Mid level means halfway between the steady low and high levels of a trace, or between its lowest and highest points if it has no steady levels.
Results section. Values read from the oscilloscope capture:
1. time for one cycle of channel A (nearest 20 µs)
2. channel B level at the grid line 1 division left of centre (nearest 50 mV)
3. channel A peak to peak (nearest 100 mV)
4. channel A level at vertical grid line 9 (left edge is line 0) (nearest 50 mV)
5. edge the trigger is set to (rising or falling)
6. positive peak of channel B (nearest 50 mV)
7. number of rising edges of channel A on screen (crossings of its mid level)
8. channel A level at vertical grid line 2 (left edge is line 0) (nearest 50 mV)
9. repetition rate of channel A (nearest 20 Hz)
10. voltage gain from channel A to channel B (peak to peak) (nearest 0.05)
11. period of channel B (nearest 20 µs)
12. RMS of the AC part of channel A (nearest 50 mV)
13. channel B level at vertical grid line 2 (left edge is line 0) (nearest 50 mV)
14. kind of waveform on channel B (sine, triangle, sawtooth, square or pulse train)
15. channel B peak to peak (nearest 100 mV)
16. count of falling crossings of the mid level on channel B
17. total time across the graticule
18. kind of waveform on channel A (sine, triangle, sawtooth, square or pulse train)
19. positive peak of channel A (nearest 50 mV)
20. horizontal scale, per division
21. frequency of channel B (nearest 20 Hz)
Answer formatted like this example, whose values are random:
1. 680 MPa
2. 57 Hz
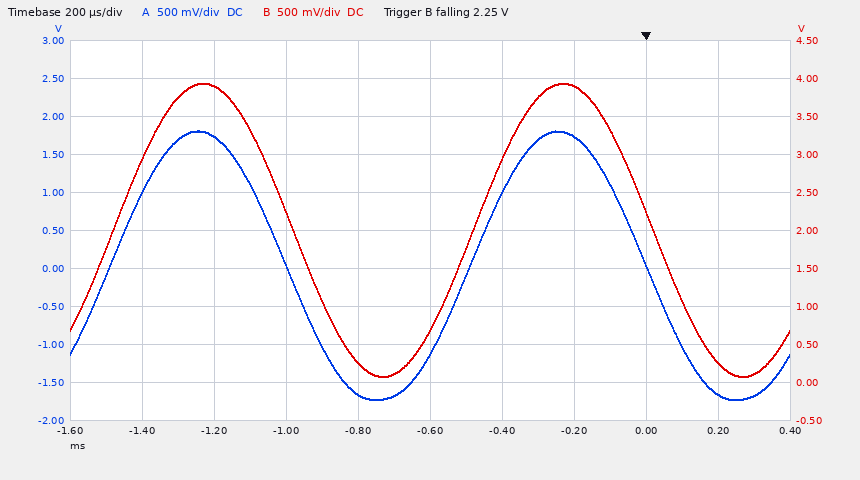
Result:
1. 1.00 ms
2. 250 mV
3. 3.50 V
4. -1.65 V
5. falling
6. 3.95 V
7. 2
8. 1.75 V
9. 1.00 kHz
10. 1.10
11. 1.00 ms
12. 1.25 V
13. 3.90 V
14. sine
15. 3.90 V
16. 2
17. 2 ms
18. sine
19. 1.80 V
20. 200 µs
21. 1.00 kHz
